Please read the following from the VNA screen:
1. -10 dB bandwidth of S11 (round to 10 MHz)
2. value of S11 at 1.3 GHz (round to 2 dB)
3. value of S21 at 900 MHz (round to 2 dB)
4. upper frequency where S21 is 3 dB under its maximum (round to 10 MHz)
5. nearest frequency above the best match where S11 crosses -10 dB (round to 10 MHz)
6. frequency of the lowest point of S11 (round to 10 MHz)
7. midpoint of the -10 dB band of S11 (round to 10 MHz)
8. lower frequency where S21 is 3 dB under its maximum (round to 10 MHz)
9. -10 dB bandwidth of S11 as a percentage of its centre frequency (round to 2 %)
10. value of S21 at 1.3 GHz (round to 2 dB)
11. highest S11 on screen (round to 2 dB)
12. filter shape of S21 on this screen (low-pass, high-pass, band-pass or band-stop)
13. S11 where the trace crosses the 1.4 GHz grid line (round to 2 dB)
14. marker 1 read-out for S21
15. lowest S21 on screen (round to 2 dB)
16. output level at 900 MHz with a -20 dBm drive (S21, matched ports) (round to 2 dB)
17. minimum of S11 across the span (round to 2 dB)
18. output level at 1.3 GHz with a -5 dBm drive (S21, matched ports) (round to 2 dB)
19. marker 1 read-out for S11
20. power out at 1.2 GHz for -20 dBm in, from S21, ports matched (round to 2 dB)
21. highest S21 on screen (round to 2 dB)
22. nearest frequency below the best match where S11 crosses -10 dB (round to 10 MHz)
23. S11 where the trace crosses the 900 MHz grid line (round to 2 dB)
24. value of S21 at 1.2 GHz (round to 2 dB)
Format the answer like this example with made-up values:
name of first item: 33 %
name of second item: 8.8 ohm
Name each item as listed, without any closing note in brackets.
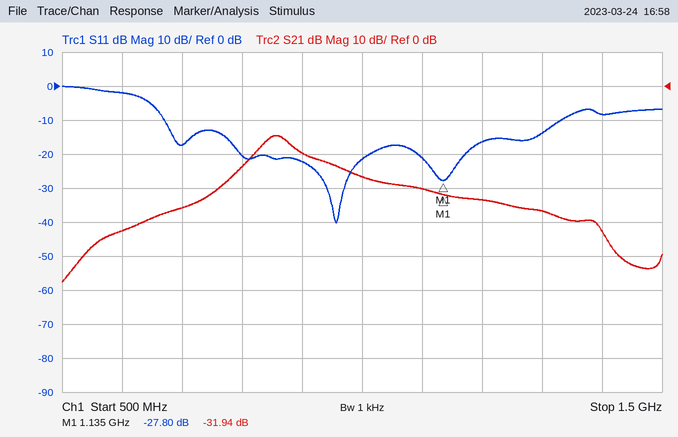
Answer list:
-10 dB bandwidth of S11: 660 MHz
value of S11 at 1.3 GHz: -14 dB
value of S21 at 900 MHz: -20 dB
upper frequency where S21 is 3 dB under its maximum: 880 MHz
nearest frequency above the best match where S11 crosses -10 dB: 1.33 GHz
frequency of the lowest point of S11: 960 MHz
midpoint of the -10 dB band of S11: 1.00 GHz
lower frequency where S21 is 3 dB under its maximum: 830 MHz
-10 dB bandwidth of S11 as a percentage of its centre frequency: 66 %
value of S21 at 1.3 GHz: -36 dB
highest S11 on screen: 0 dB
filter shape of S21 on this screen: band-pass
S11 where the trace crosses the 1.4 GHz grid line: -8 dB
marker 1 read-out for S21: -31.94 dB
lowest S21 on screen: -58 dB
output level at 900 MHz with a -20 dBm drive (S21, matched ports): -40 dBm
minimum of S11 across the span: -40 dB
output level at 1.3 GHz with a -5 dBm drive (S21, matched ports): -42 dBm
marker 1 read-out for S11: -27.80 dB
power out at 1.2 GHz for -20 dBm in, from S21, ports matched: -54 dBm
highest S21 on screen: -14 dB
nearest frequency below the best match where S11 crosses -10 dB: 670 MHz
S11 where the trace crosses the 900 MHz grid line: -22 dB
value of S21 at 1.2 GHz: -34 dB
